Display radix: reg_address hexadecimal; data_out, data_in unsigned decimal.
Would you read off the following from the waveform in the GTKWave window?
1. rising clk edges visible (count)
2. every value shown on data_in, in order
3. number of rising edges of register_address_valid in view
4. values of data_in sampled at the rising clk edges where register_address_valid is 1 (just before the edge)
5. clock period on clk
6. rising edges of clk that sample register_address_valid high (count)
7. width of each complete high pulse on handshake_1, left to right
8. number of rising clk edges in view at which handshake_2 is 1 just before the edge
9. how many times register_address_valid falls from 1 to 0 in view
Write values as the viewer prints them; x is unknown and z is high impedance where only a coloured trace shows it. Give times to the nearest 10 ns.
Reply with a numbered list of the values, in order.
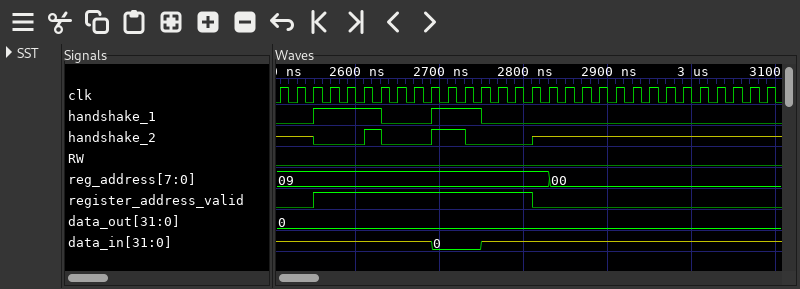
1. 30
2. z, 0, z
3. 1
4. z, z, z, z, z, z, z, 0, 0, 0, z, z, z
5. 20 ns
6. 13
7. 80 ns, 60 ns
8. 3
9. 1
